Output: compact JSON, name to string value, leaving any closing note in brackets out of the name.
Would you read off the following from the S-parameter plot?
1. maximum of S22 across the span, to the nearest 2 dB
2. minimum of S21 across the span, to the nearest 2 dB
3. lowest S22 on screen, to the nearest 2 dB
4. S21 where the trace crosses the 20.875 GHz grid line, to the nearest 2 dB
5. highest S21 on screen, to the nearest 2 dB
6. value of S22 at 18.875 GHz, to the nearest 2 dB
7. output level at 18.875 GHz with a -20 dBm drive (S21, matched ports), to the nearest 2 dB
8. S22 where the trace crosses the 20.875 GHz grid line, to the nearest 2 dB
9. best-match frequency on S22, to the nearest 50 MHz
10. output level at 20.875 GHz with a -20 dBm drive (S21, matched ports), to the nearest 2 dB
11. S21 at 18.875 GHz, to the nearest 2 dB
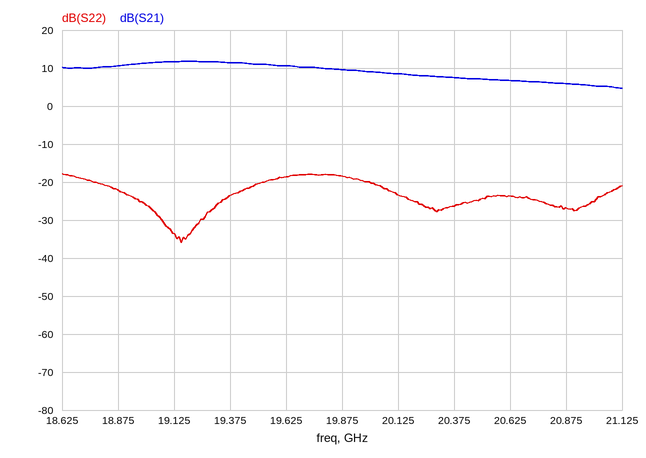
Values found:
{"maximum of S22 across the span, to the nearest 2 dB": "-18 dB", "minimum of S21 across the span, to the nearest 2 dB": "4 dB", "lowest S22 on screen, to the nearest 2 dB": "-36 dB", "S21 where the trace crosses the 20.875 GHz grid line, to the nearest 2 dB": "6 dB", "highest S21 on screen, to the nearest 2 dB": "12 dB", "value of S22 at 18.875 GHz, to the nearest 2 dB": "-22 dB", "output level at 18.875 GHz with a -20 dBm drive (S21, matched ports), to the nearest 2 dB": "-10 dBm", "S22 where the trace crosses the 20.875 GHz grid line, to the nearest 2 dB": "-26 dB", "best-match frequency on S22, to the nearest 50 MHz": "19.15 GHz", "output level at 20.875 GHz with a -20 dBm drive (S21, matched ports), to the nearest 2 dB": "-14 dBm", "S21 at 18.875 GHz, to the nearest 2 dB": "10 dB"}
